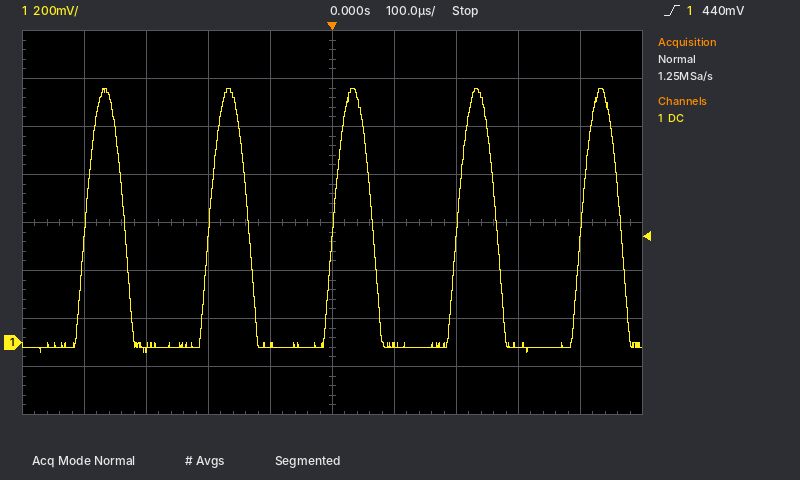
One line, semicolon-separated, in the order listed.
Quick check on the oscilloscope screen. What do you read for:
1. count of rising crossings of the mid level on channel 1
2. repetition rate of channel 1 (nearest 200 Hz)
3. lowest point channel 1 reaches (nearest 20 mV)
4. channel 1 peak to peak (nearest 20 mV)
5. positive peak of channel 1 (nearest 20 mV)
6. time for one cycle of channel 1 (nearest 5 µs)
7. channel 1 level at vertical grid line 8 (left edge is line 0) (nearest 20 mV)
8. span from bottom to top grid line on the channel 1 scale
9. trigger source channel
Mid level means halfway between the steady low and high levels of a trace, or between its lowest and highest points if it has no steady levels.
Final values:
5; 5.0 kHz; -40 mV; 1.10 V; 1.06 V; 200 µs; -20 mV; 1.6 V; channel 1
